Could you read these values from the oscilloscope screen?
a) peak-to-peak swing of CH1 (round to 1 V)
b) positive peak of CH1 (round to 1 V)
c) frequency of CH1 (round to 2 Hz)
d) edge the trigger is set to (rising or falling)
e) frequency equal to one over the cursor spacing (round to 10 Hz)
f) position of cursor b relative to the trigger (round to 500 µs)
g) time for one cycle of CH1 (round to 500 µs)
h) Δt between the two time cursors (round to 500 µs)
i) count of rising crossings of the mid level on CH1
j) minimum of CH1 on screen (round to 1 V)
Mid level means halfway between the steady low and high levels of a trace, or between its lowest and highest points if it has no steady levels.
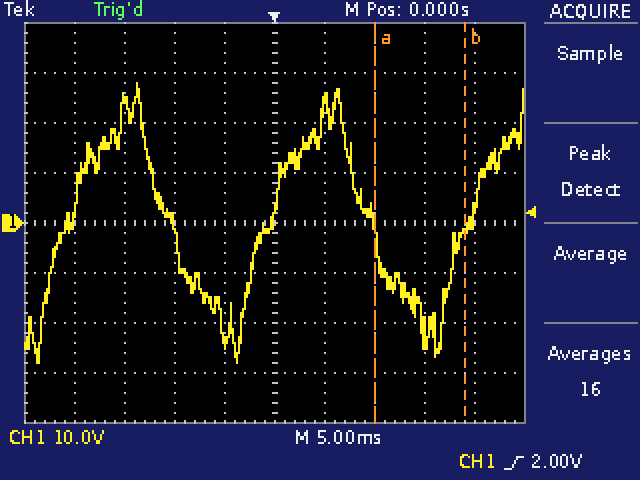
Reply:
56 V
28 V
50 Hz
rising
110 Hz
+19.0 ms
20.0 ms
9.0 ms
3
-28 V
